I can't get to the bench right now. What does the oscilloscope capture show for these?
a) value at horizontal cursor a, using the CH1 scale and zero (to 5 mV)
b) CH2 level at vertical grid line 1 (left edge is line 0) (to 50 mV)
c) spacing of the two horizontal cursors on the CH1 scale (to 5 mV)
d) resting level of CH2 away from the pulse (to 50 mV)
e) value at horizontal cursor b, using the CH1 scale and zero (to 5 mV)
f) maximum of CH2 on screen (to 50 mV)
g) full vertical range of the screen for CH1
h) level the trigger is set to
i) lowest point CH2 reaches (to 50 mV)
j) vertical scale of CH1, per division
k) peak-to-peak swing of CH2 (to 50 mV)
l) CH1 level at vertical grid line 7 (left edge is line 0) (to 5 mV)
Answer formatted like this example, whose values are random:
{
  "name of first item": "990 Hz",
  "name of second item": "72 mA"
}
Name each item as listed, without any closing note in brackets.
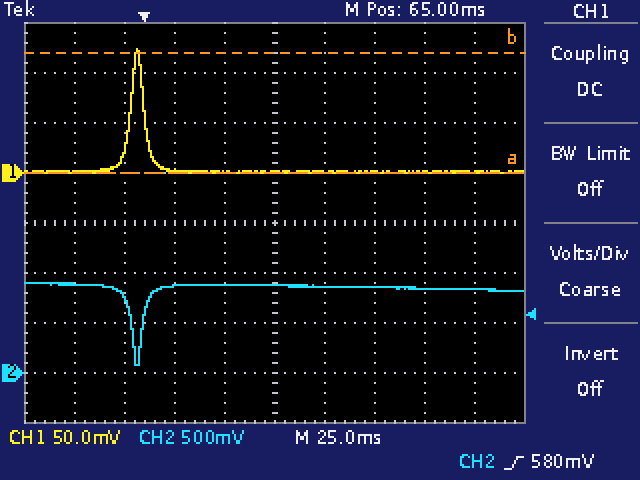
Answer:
{
  "value at horizontal cursor a, using the CH1 scale and zero": "0 mV",
  "CH2 level at vertical grid line 1 (left edge is line 0)": "900 mV",
  "spacing of the two horizontal cursors on the CH1 scale": "120 mV",
  "resting level of CH2 away from the pulse": "850 mV",
  "value at horizontal cursor b, using the CH1 scale and zero": "120 mV",
  "maximum of CH2 on screen": "900 mV",
  "full vertical range of the screen for CH1": "400 mV",
  "level the trigger is set to": "580 mV",
  "lowest point CH2 reaches": "100 mV",
  "vertical scale of CH1, per division": "50 mV",
  "peak-to-peak swing of CH2": "800 mV",
  "CH1 level at vertical grid line 7 (left edge is line 0)": "0 mV"
}
